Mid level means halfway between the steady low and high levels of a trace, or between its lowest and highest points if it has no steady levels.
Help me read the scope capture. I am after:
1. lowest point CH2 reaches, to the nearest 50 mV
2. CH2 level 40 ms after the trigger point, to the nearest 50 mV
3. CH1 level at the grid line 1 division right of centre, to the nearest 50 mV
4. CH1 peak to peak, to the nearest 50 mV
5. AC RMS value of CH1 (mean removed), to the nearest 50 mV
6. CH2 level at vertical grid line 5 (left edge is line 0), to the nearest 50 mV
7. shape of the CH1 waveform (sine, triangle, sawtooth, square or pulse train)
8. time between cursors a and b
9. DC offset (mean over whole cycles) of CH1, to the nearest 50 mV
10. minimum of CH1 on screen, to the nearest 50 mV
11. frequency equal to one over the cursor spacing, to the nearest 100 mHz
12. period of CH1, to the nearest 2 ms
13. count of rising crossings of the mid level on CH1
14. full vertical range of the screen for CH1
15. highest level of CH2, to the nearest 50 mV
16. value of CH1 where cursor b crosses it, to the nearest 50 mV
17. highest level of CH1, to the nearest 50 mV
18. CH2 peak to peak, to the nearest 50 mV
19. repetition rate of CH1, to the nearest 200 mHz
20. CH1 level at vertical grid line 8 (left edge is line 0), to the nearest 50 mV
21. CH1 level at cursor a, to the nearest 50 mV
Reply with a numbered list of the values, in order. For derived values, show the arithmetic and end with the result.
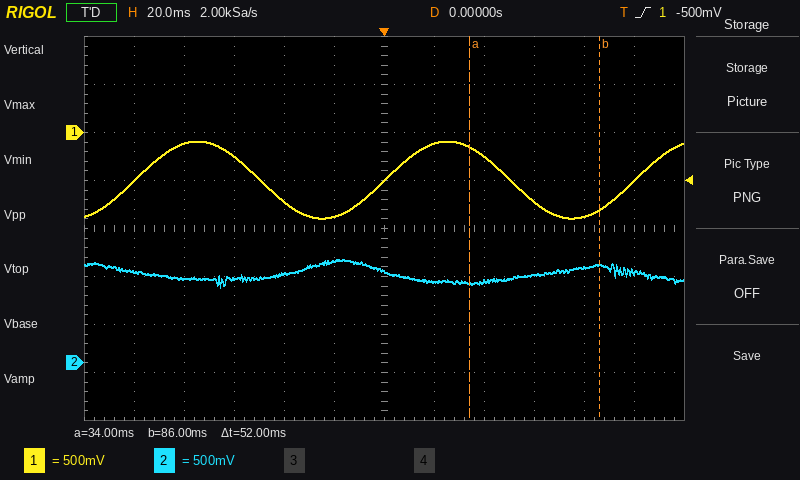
1. 800 mV
2. 850 mV
3. -100 mV
4. -100 mV − (-900 mV) = 800 mV
5. 800 mV / (2√2) ≈ 283 mV, so 300 mV to the nearest 50 mV
6. 1.05 V
7. sine
8. 52 ms
9. (-100 mV + (-900 mV)) / 2 ≈ -500 mV
10. -900 mV
11. 1 / 52 ms ≈ 19.2 Hz
12. 100 ms
13. 3
14. 4 V
15. 1.10 V
16. -800 mV
17. -100 mV
18. 1.10 V − (800 mV) = 300 mV
19. 1 / 100 ms ≈ 10.0 Hz
20. -250 mV
21. -150 mV
